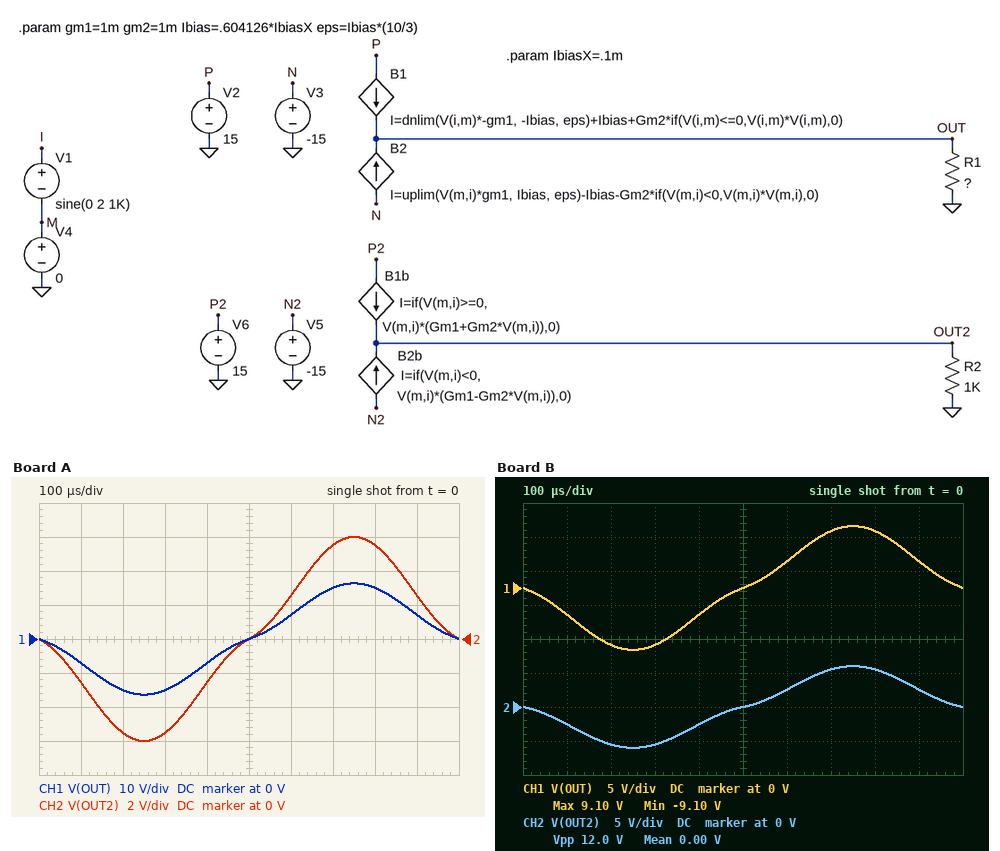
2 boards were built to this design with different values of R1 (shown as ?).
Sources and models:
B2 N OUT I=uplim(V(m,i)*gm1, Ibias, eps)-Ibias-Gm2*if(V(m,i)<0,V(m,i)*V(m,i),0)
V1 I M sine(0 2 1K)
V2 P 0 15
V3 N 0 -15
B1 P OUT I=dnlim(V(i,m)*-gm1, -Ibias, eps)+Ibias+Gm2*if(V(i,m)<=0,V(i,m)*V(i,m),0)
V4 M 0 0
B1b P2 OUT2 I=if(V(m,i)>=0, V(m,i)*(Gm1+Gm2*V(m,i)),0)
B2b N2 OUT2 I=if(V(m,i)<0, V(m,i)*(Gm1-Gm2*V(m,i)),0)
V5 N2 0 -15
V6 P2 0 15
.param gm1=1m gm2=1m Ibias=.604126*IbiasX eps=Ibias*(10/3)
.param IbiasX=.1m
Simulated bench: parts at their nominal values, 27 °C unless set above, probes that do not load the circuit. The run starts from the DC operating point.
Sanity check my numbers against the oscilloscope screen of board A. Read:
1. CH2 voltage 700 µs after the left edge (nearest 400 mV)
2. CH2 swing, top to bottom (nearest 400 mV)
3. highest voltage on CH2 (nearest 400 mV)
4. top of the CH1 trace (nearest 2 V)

5.6 V
12.0 V
6.0 V
16 V
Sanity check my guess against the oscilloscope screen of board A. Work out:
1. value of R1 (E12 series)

2.7 kΩ
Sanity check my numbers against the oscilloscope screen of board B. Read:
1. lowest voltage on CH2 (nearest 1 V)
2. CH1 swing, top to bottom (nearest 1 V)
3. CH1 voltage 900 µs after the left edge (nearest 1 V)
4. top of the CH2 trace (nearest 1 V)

-6 V
18 V
4 V
6 V
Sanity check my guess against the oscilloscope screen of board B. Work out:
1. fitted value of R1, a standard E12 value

1.5 kΩ
